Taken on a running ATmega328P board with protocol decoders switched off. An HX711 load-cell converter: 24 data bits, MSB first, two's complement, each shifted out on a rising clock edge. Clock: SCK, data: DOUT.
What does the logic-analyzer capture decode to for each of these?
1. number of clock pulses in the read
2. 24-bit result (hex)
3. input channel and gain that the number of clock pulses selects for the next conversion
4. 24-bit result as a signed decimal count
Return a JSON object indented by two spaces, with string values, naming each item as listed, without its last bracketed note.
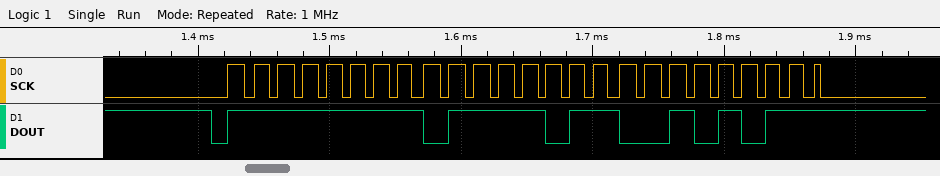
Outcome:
{
  "number of clock pulses in the read": "25",
  "24-bit result": "0xFF7B2B",
  "input channel and gain that the number of clock pulses selects for the next conversion": "channel A, gain 128",
  "24-bit result as a signed decimal count": "-34005"
}
